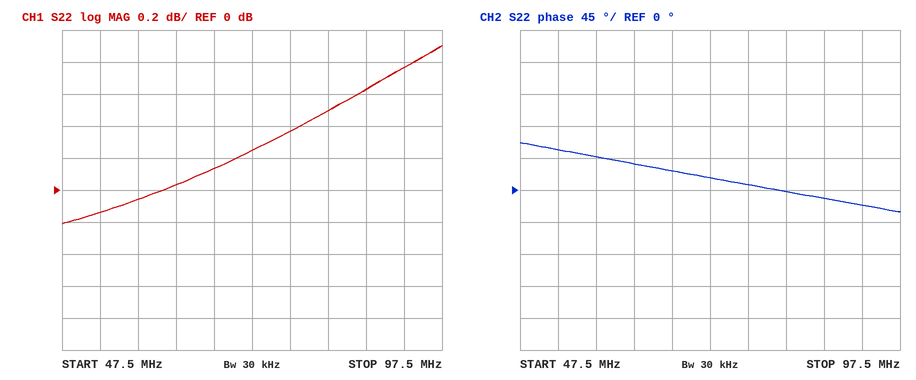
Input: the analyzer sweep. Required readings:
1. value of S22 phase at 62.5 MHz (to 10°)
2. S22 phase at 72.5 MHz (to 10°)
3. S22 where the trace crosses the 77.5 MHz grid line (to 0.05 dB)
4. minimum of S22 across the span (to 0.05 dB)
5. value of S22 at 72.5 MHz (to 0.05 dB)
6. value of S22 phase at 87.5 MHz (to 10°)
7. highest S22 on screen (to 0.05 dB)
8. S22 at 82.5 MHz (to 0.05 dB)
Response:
40°
20°
0.35 dB
-0.20 dB
0.25 dB
-10°
0.90 dB
0.50 dB
